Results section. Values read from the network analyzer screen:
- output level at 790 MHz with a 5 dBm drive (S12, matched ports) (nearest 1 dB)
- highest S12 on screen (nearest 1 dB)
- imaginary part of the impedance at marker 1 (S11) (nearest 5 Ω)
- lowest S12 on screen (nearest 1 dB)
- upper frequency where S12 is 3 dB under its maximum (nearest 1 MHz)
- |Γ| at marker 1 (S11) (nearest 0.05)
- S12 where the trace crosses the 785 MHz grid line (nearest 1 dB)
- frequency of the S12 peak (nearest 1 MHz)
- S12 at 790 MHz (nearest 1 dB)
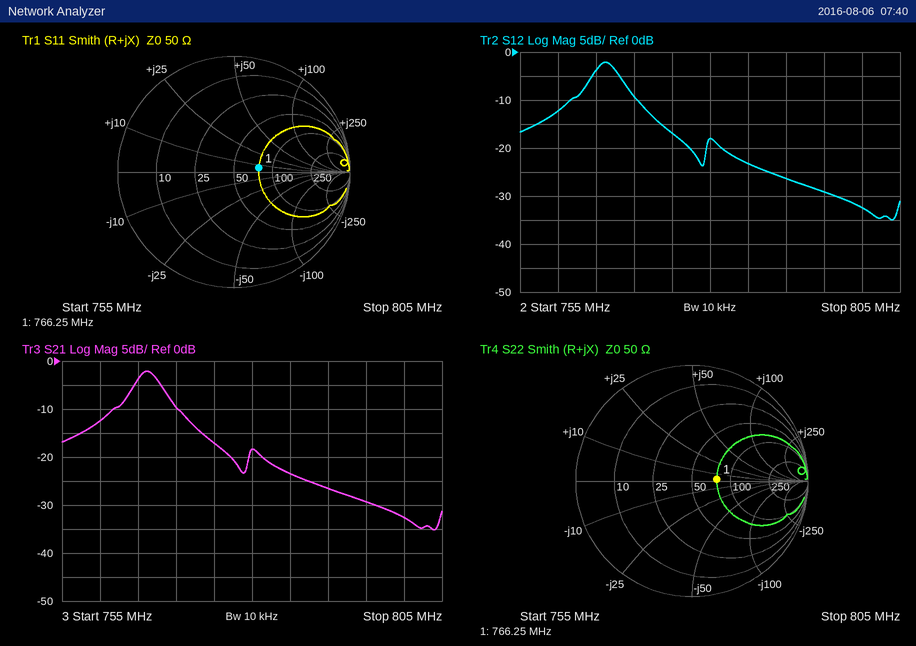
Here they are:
-21 dBm
-2 dB
+5 Ω
-35 dB
768 MHz
0.20
-23 dB
766 MHz
-26 dB
